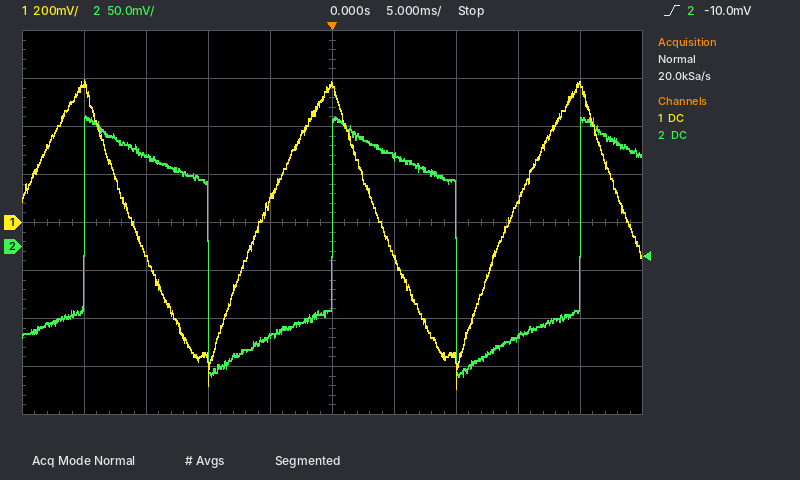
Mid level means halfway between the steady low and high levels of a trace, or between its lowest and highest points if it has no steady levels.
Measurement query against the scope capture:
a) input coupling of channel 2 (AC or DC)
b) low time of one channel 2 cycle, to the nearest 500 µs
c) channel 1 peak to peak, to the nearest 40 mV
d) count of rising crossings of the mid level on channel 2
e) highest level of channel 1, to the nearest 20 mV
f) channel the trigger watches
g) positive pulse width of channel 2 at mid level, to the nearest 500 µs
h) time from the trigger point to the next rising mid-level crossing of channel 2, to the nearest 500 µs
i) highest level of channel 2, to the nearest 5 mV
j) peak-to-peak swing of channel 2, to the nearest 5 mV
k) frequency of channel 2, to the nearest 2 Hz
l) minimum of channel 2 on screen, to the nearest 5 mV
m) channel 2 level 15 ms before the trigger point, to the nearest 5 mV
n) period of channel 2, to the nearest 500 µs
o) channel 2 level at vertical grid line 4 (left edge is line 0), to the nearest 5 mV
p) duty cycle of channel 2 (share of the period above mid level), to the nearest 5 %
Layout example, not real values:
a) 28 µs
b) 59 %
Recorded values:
a) DC
b) 10.0 ms
c) 1.28 V
d) 3
e) 600 mV
f) channel 2
g) 10.0 ms
h) 20.0 ms
i) 135 mV
j) 270 mV
k) 50 Hz
l) -135 mV
m) 95 mV
n) 20.0 ms
o) -95 mV
p) 50 %
